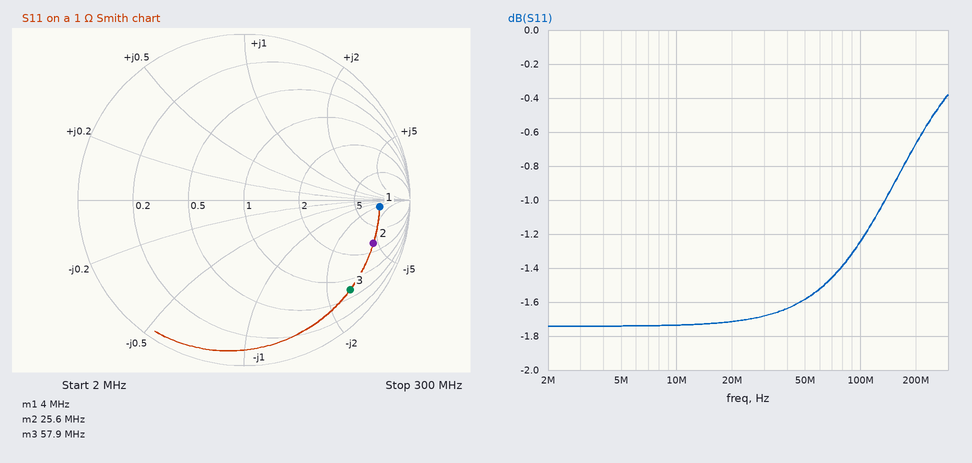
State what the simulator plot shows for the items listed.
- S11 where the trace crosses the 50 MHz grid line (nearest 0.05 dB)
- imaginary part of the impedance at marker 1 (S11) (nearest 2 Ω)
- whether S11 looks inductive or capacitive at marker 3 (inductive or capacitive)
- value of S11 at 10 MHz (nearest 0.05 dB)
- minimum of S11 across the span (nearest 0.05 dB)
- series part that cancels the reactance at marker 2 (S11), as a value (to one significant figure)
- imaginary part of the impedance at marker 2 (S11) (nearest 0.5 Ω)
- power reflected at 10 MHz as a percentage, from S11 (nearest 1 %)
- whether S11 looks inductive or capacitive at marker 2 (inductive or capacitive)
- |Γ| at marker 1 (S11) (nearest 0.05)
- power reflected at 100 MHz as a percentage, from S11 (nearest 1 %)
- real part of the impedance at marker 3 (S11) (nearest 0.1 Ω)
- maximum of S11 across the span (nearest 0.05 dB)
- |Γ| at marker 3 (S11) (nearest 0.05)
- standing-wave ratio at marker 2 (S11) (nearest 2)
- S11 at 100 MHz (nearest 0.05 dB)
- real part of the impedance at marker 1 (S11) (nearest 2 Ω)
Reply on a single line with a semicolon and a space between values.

-1.60 dB; -2 Ω; capacitive; -1.75 dB; -1.75 dB; 30 nH; -4.5 Ω; 67 %; capacitive; 0.80; 75 %; 0.7 Ω; -0.40 dB; 0.85; 10; -1.25 dB; 10 Ω
